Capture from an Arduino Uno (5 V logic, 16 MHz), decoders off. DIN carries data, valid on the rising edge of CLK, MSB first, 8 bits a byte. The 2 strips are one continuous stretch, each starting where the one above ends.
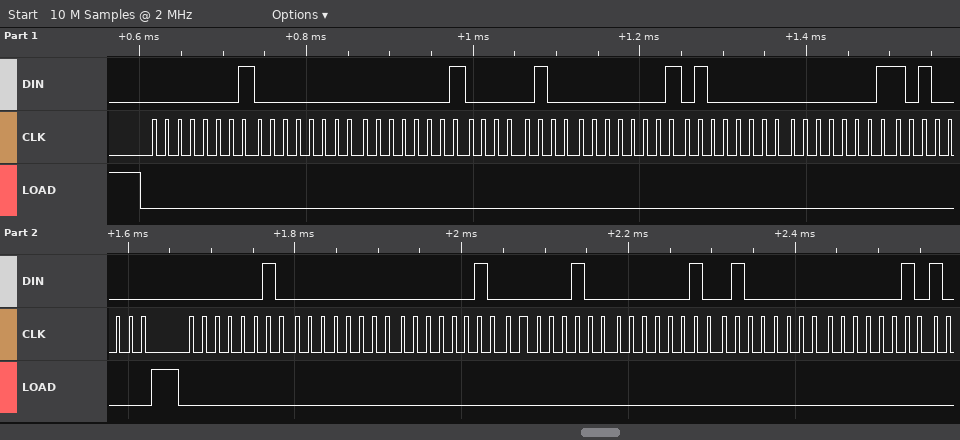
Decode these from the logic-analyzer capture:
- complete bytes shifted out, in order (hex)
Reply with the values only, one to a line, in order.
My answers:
01 00 01 04 01 40 01 A0 02 00 02 04 02 40 02
